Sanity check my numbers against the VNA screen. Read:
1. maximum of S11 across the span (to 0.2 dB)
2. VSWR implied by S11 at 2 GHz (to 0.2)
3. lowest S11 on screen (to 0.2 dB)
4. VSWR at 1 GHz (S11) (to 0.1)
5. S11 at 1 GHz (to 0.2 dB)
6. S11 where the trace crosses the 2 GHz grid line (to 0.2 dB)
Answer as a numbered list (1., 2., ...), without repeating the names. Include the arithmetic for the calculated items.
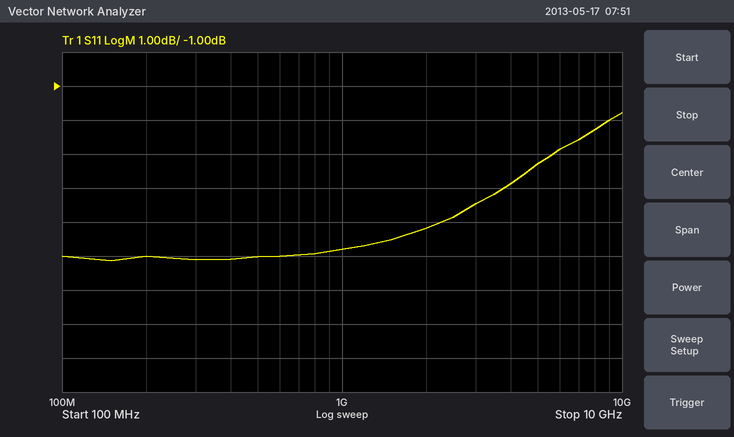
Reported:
1. -1.8 dB
2. |Γ| = 10^(-5.2/20) = 0.5495; VSWR = (1 + 0.5495)/(1 − 0.5495) ≈ 3.4
3. -6.2 dB
4. |Γ| = 10^(-5.8/20) = 0.5129; VSWR = (1 + 0.5129)/(1 − 0.5129) ≈ 3.1
5. -5.8 dB
6. -5.2 dB
